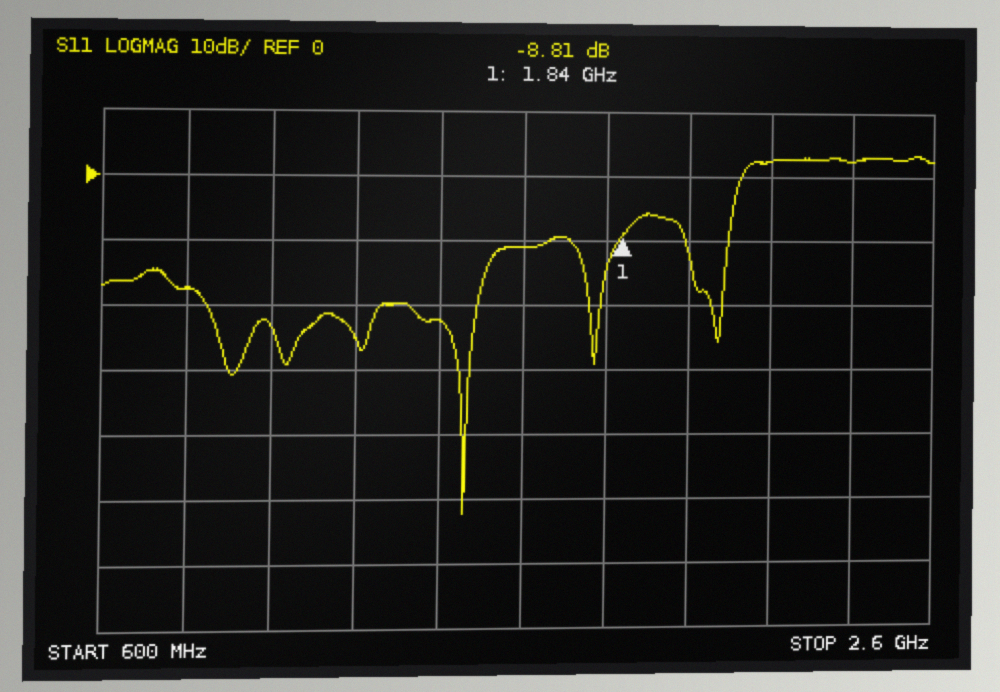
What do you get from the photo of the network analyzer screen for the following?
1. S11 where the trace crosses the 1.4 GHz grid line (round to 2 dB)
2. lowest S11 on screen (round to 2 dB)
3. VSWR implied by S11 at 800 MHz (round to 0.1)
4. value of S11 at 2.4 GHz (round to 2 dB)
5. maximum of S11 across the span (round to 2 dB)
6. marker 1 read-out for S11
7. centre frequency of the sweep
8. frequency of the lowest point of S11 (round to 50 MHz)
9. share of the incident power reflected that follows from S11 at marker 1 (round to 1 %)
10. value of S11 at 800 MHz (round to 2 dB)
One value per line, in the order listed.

-22 dB
-52 dB
1.3
2 dB
4 dB
-8.81 dB
1.6 GHz
1.45 GHz
13 %
-18 dB
